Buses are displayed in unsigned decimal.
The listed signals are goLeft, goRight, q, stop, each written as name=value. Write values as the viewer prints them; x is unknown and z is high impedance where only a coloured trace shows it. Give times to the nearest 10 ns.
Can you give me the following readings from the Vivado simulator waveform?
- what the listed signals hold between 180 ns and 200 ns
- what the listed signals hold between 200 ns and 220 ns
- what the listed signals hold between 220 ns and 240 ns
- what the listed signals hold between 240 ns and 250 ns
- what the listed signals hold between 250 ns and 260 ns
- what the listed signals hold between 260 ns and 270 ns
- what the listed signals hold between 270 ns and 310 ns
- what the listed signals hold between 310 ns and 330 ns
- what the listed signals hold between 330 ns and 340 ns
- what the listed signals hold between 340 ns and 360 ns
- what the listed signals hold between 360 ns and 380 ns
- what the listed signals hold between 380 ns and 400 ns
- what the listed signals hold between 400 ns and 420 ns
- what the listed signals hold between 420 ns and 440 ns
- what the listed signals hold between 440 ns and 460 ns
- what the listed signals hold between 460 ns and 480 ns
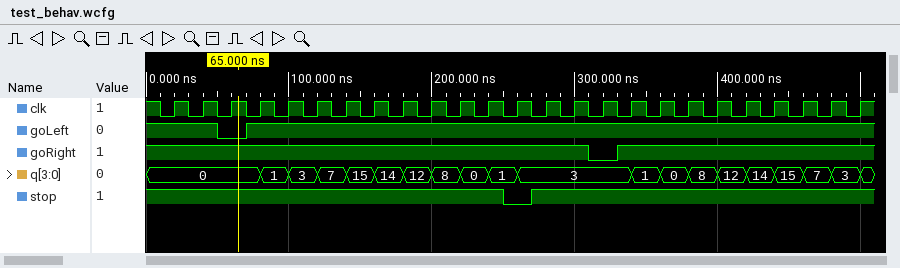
goLeft=1, goRight=1, q=12, stop=1
goLeft=1, goRight=1, q=8, stop=1
goLeft=1, goRight=1, q=0, stop=1
goLeft=1, goRight=1, q=1, stop=1
goLeft=1, goRight=1, q=1, stop=0
goLeft=1, goRight=1, q=3, stop=0
goLeft=1, goRight=1, q=3, stop=1
goLeft=1, goRight=0, q=3, stop=1
goLeft=1, goRight=1, q=3, stop=1
goLeft=1, goRight=1, q=1, stop=1
goLeft=1, goRight=1, q=0, stop=1
goLeft=1, goRight=1, q=8, stop=1
goLeft=1, goRight=1, q=12, stop=1
goLeft=1, goRight=1, q=14, stop=1
goLeft=1, goRight=1, q=15, stop=1
goLeft=1, goRight=1, q=7, stop=1
